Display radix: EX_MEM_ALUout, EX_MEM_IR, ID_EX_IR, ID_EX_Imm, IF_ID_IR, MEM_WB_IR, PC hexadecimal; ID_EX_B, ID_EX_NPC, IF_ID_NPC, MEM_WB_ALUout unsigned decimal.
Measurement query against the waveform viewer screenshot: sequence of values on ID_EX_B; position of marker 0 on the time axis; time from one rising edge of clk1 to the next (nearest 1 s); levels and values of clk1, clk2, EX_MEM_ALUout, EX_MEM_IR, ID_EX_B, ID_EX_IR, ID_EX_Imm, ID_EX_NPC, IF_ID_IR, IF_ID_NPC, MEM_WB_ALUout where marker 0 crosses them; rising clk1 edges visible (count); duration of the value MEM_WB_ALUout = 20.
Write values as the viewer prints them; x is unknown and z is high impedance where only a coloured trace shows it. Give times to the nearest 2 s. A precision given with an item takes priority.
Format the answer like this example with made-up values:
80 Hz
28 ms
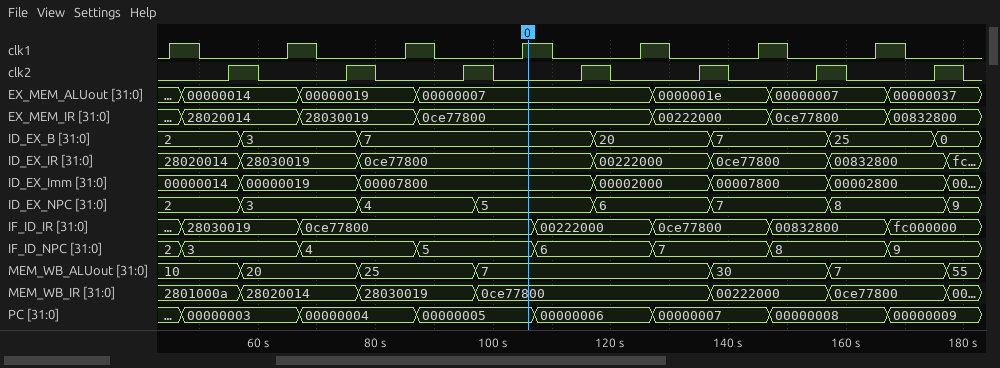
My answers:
2, 3, 7, 20, 7, 25, 0
106 s
20 s
clk1=1, clk2=0, EX_MEM_ALUout=00000007, EX_MEM_IR=0ce77800, ID_EX_B=7, ID_EX_IR=0ce77800, ID_EX_Imm=00007800, ID_EX_NPC=5, IF_ID_IR=0ce77800, IF_ID_NPC=5, MEM_WB_ALUout=7
7
20 s
